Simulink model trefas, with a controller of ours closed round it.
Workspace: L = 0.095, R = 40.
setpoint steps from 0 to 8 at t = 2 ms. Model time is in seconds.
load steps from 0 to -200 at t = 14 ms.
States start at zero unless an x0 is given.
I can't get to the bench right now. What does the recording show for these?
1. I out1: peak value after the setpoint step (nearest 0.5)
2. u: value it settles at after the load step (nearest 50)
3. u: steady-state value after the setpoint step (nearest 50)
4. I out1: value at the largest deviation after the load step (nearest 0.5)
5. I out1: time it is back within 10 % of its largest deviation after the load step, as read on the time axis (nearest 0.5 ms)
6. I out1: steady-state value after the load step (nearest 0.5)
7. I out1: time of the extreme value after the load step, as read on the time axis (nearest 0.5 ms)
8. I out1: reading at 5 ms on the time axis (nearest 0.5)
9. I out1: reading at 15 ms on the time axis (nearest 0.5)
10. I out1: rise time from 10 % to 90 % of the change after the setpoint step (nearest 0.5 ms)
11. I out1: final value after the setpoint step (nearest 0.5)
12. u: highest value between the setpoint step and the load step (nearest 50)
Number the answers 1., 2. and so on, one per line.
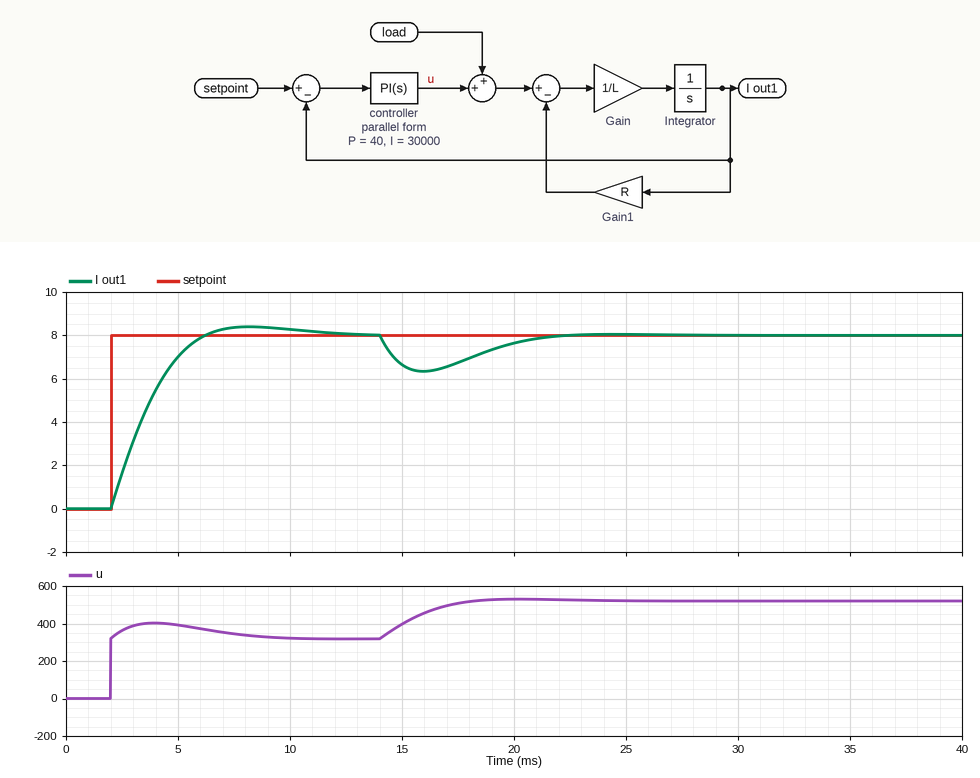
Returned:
1. 8.5
2. 500
3. 300
4. 6.5
5. 21.0 ms
6. 8.0
7. 16.0 ms
8. 7.0
9. 6.5
10. 3.0 ms
11. 8.0
12. 400
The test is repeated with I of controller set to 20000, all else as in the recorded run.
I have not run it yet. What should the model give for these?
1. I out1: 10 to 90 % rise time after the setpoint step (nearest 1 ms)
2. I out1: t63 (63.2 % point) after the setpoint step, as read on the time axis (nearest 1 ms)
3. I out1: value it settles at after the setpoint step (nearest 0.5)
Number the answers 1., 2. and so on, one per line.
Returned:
1. 4 ms
2. 4 ms
3. 8.0
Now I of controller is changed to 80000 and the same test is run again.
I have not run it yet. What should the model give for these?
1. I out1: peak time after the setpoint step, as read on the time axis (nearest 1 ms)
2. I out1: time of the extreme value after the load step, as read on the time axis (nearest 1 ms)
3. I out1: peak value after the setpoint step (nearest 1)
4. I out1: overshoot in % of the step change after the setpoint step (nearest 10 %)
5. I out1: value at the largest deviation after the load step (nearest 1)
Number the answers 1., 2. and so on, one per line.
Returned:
1. 5 ms
2. 15 ms
3. 10
4. 20 %
5. 7
